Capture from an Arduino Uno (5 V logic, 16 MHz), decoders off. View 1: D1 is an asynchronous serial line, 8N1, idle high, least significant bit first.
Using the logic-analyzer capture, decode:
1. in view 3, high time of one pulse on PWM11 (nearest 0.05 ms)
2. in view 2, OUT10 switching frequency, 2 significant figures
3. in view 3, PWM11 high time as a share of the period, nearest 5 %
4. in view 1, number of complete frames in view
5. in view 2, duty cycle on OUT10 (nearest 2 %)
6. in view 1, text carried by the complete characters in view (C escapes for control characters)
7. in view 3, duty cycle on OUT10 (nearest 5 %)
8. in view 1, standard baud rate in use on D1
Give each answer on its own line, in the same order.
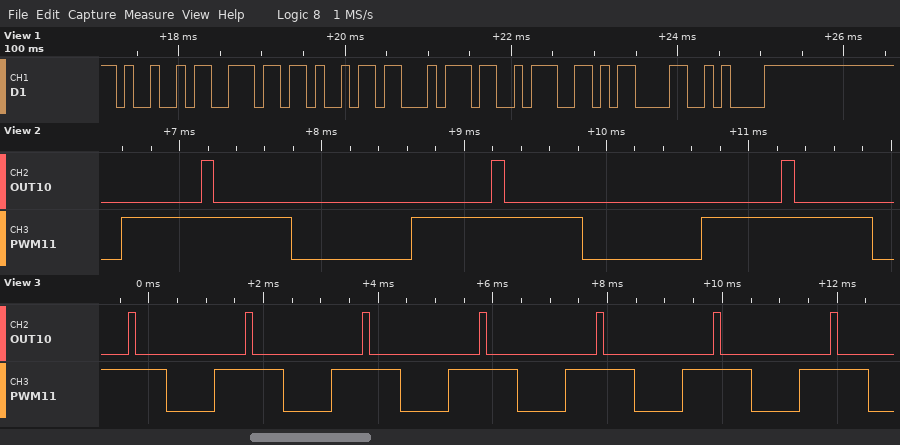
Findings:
1.20 ms
490 Hz
60 %
7
4 %
"Init:\r\n"
5 %
9600 baud
